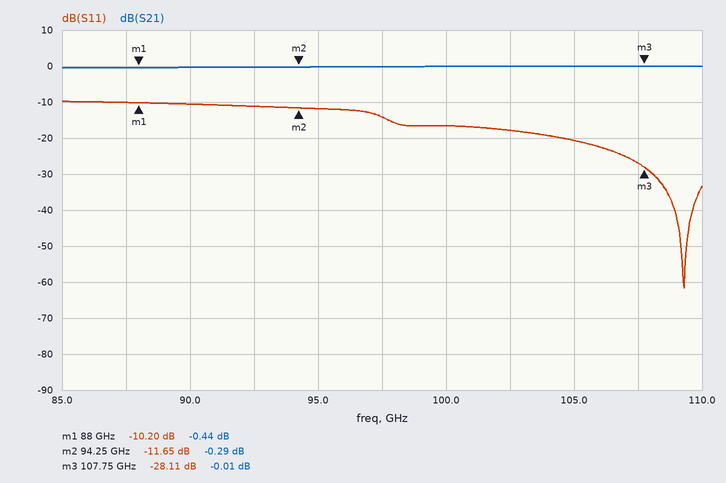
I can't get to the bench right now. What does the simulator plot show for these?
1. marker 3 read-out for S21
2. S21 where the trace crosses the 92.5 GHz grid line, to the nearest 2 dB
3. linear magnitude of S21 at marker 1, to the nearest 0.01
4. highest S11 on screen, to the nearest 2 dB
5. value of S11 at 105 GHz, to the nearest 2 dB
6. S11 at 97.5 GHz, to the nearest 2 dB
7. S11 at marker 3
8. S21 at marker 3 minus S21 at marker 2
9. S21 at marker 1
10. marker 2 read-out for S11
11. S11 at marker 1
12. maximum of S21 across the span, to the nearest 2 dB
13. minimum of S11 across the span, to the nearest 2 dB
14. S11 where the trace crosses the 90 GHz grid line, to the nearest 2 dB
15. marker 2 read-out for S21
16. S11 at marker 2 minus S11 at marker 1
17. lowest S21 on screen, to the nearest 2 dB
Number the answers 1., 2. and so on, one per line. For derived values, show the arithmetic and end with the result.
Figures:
1. -0.01 dB
2. 0 dB
3. 10^(-0.44/20) ≈ 0.95
4. -10 dB
5. -20 dB
6. -14 dB
7. -28.11 dB
8. -0.01 − (-0.29) = 0.28 dB
9. -0.44 dB
10. -11.65 dB
11. -10.20 dB
12. 0 dB
13. -62 dB
14. -10 dB
15. -0.29 dB
16. -11.65 − (-10.2) = -1.45 dB
17. 0 dB
